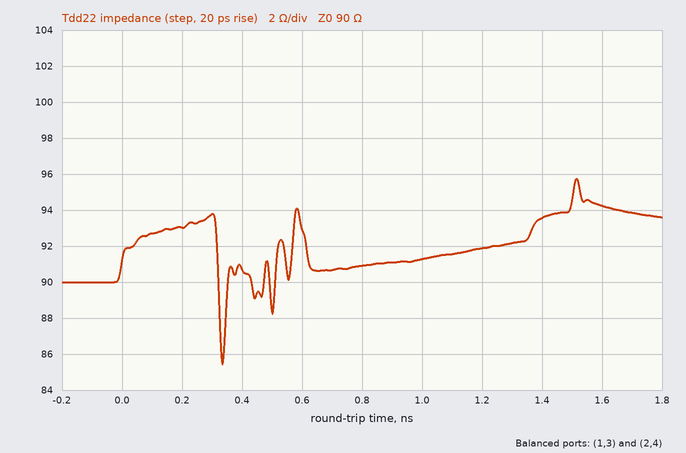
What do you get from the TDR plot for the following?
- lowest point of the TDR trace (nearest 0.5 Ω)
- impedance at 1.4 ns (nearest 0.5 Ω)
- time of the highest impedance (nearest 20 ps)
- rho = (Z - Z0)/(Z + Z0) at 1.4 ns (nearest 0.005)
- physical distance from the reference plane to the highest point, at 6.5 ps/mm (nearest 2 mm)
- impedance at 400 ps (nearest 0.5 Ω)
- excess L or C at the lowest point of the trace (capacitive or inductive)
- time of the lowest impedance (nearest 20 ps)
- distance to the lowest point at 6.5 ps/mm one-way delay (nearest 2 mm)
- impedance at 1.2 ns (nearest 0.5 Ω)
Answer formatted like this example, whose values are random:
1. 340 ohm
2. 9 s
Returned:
1. 85.5 Ω
2. 93.5 Ω
3. 1.52 ns
4. +0.020
5. 116 mm
6. 90.5 Ω
7. capacitive
8. 340 ps
9. 26 mm
10. 92.0 Ω
